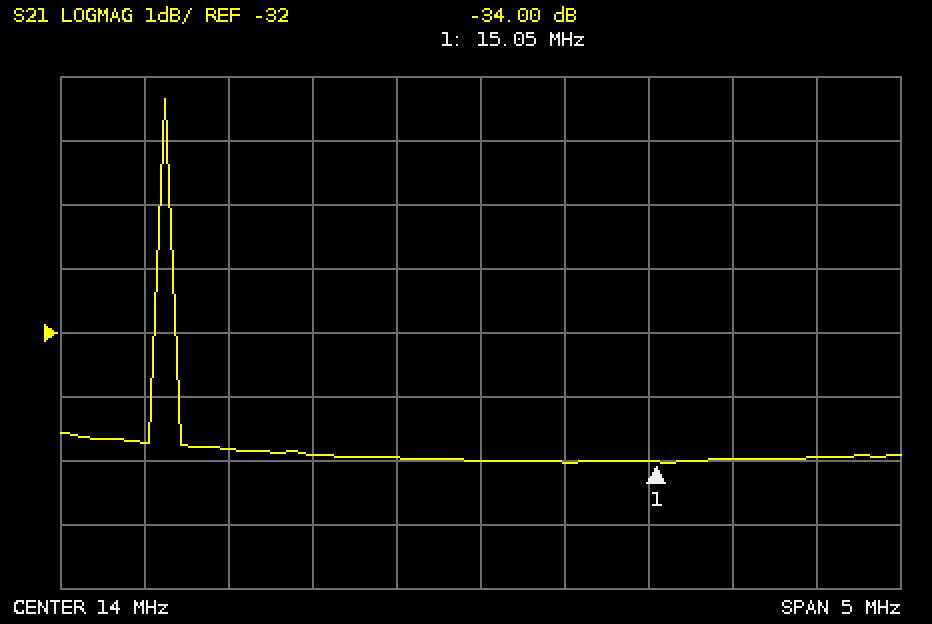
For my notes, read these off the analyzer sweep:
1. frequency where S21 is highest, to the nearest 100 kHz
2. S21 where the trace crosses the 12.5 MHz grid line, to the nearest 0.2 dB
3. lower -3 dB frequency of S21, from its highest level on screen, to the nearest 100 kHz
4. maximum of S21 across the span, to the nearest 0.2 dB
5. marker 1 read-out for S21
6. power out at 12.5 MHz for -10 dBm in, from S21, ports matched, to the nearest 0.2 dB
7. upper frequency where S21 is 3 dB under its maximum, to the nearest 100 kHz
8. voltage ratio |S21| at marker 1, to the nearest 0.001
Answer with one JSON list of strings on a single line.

["12.1 MHz", "-33.8 dB", "12.1 MHz", "-28.4 dB", "-34.00 dB", "-43.8 dBm", "12.2 MHz", "0.020"]
